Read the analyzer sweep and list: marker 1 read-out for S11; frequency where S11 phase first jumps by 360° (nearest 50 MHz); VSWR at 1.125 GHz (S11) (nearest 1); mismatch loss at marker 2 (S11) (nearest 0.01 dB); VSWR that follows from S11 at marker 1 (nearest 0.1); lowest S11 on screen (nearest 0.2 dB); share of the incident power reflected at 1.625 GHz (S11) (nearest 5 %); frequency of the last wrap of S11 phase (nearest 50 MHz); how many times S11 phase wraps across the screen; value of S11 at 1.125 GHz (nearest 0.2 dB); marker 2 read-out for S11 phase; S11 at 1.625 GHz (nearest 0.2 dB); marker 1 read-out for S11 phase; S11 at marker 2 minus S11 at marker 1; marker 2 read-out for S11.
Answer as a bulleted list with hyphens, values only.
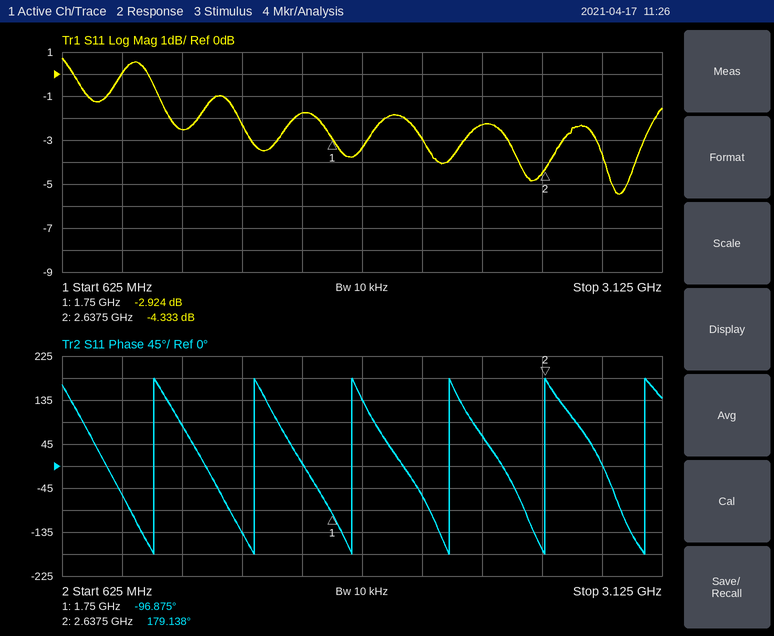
- -2.924 dB
- 1.00 GHz
- 7
- 2.00 dB
- 6.0
- -5.4 dB
- 65 %
- 3.05 GHz
- 6
- -2.6 dB
- 179.138°
- -1.8 dB
- -96.875°
- -1.409 dB
- -4.333 dB
